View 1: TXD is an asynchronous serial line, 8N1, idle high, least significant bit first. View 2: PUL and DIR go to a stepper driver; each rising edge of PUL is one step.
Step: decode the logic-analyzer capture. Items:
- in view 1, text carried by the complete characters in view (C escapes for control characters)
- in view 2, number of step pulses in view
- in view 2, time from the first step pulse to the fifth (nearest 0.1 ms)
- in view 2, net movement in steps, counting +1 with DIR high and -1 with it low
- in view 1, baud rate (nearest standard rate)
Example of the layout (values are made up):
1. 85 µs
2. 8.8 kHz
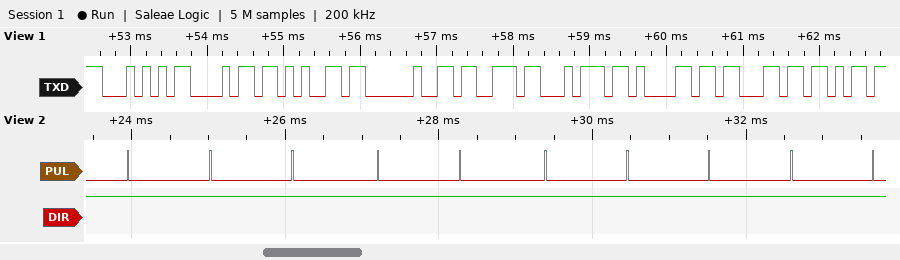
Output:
1. "The stack"
2. 10
3. 4.3 ms
4. +10
5. 9600 baud
